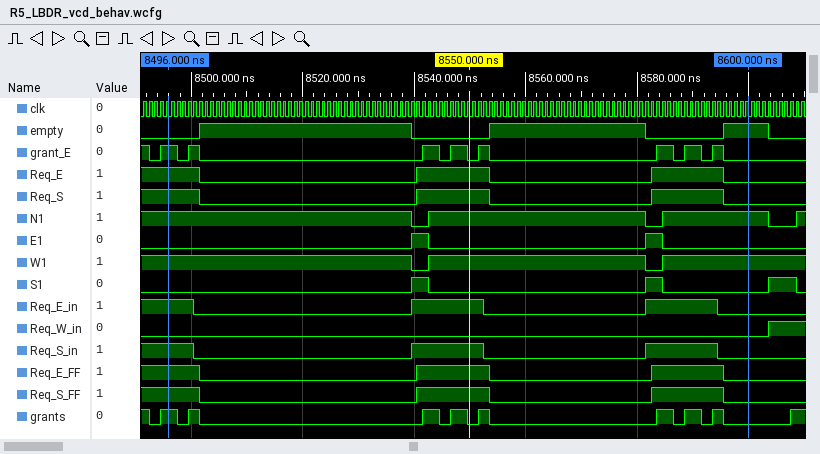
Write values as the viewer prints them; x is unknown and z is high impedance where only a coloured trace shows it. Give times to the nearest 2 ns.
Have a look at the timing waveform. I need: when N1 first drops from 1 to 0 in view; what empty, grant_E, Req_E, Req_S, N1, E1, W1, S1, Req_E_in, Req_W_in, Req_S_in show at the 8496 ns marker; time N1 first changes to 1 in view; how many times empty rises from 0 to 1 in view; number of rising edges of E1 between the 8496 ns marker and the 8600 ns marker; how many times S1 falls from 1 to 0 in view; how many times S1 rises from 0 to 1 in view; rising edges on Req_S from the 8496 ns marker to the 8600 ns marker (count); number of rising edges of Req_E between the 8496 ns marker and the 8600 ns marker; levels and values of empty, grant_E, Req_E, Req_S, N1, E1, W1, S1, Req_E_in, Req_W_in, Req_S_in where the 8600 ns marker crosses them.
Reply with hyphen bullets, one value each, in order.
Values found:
- 8540 ns
- empty=0, grant_E=1, Req_E=1, Req_S=1, N1=1, E1=0, W1=1, S1=0, Req_E_in=1, Req_W_in=0, Req_S_in=1
- 8542 ns
- 3
- 2
- 3
- 3
- 2
- 2
- empty=1, grant_E=0, Req_E=0, Req_S=0, N1=1, E1=0, W1=1, S1=0, Req_E_in=0, Req_W_in=0, Req_S_in=0
